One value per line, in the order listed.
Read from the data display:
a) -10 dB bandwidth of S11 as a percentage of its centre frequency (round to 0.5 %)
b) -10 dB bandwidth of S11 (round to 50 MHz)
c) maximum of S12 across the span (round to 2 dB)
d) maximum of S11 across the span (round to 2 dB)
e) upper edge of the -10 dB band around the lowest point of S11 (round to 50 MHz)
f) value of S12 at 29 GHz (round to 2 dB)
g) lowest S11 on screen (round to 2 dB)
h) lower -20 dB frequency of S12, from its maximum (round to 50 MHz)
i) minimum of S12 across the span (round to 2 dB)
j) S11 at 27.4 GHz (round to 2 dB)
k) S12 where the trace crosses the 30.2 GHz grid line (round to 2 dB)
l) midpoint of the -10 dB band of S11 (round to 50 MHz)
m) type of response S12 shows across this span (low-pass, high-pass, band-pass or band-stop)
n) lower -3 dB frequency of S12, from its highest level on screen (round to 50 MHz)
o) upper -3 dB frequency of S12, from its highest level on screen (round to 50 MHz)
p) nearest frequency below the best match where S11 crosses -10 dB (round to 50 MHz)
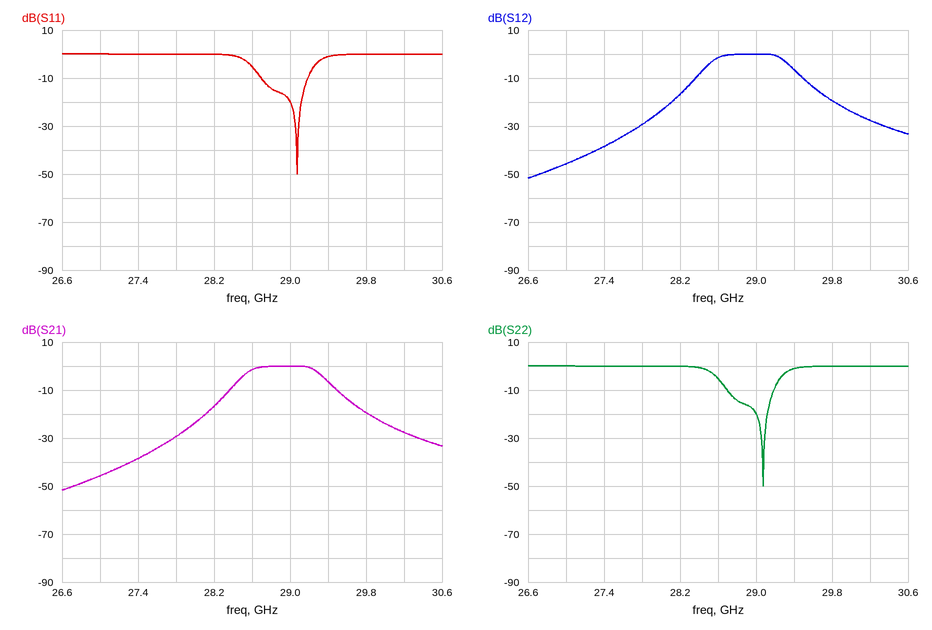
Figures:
1.5 %
500 MHz
0 dB
0 dB
29.20 GHz
0 dB
-50 dB
28.10 GHz
-52 dB
0 dB
-28 dB
28.95 GHz
band-pass
28.55 GHz
29.30 GHz
28.70 GHz
